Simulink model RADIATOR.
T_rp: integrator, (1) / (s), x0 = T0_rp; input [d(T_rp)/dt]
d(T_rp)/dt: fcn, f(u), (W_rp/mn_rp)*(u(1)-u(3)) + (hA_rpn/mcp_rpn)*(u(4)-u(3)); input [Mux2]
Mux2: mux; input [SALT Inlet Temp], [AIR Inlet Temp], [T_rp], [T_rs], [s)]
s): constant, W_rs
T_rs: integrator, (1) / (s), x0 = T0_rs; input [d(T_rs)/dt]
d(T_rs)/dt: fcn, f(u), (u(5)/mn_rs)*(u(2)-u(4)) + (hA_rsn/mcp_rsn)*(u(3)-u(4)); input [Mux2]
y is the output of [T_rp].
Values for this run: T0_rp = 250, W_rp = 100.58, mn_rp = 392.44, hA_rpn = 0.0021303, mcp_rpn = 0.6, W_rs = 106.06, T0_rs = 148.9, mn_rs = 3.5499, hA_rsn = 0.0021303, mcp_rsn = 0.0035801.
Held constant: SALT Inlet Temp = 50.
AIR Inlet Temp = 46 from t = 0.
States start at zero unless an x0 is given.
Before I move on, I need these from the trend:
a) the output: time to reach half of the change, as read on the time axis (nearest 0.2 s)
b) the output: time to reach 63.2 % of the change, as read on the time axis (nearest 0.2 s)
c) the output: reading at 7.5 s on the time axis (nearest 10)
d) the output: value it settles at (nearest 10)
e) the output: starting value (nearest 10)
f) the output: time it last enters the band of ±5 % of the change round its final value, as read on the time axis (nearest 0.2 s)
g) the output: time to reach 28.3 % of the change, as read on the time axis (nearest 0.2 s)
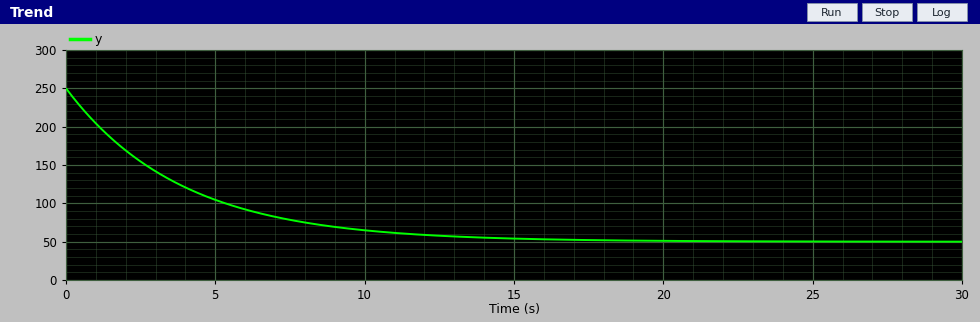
2.6 s
3.8 s
80
50
250
11.6 s
1.2 s
